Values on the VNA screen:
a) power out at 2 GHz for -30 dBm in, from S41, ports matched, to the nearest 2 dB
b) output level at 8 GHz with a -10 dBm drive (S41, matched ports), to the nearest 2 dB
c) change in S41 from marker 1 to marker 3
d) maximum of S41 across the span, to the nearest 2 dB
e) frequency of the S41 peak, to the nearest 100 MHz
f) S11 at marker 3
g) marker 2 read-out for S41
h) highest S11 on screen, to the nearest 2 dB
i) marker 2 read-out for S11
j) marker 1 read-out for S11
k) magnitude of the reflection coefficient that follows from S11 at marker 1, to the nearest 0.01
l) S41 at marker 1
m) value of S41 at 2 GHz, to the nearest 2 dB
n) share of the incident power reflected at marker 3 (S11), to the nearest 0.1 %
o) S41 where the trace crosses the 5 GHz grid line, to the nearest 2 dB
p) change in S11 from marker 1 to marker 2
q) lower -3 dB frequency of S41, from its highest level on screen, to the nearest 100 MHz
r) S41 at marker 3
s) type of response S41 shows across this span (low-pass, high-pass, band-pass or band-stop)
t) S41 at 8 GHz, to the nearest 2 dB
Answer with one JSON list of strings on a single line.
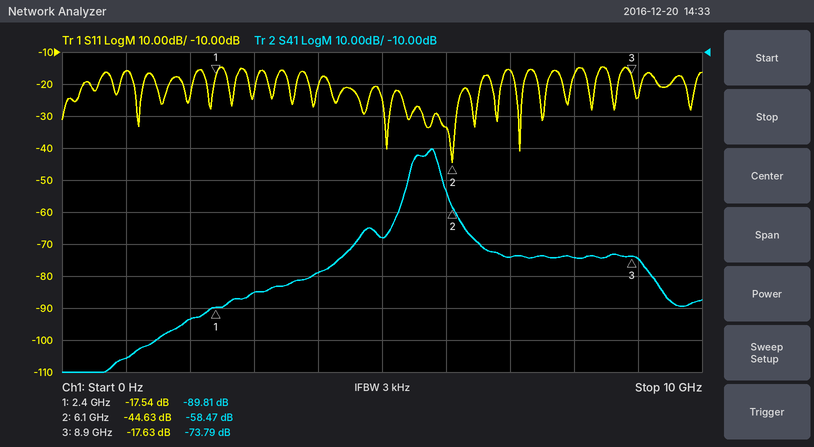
["-124 dBm", "-84 dBm", "16.02 dB", "-40 dB", "5.8 GHz", "-17.63 dB", "-58.47 dB", "-14 dB", "-44.63 dB", "-17.54 dB", "0.13", "-89.81 dB", "-94 dB", "1.7 %", "-68 dB", "-27.09 dB", "5.5 GHz", "-73.79 dB", "band-pass", "-74 dB"]
